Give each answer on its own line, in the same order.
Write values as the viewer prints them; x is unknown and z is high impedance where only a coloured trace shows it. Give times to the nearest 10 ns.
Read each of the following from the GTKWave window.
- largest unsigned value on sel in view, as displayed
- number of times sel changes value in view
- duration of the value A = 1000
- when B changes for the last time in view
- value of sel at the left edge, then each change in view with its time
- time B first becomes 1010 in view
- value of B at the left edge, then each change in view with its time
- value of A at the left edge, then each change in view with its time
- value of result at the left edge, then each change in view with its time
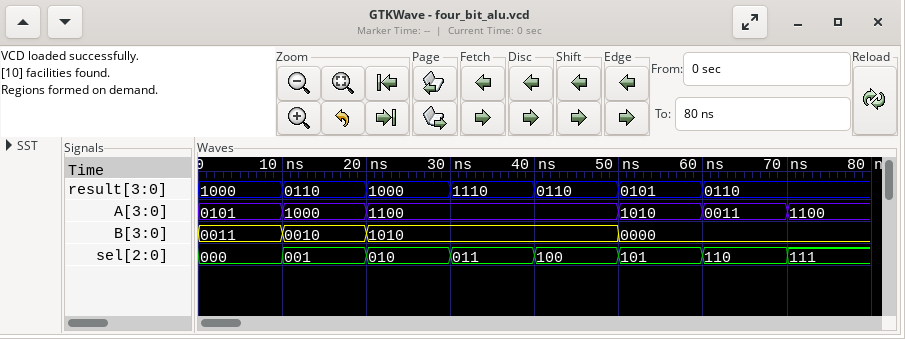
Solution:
111
7
10 ns
50 ns
000, 001 at 10 ns, 010 at 20 ns, 011 at 30 ns, 100 at 40 ns, 101 at 50 ns, 110 at 60 ns, 111 at 70 ns
20 ns
0011, 0010 at 10 ns, 1010 at 20 ns, 0000 at 50 ns
0101, 1000 at 10 ns, 1100 at 20 ns, 1010 at 50 ns, 0011 at 60 ns, 1100 at 70 ns
1000, 0110 at 10 ns, 1000 at 20 ns, 1110 at 30 ns, 0110 at 40 ns, 0101 at 50 ns, 0110 at 60 ns
